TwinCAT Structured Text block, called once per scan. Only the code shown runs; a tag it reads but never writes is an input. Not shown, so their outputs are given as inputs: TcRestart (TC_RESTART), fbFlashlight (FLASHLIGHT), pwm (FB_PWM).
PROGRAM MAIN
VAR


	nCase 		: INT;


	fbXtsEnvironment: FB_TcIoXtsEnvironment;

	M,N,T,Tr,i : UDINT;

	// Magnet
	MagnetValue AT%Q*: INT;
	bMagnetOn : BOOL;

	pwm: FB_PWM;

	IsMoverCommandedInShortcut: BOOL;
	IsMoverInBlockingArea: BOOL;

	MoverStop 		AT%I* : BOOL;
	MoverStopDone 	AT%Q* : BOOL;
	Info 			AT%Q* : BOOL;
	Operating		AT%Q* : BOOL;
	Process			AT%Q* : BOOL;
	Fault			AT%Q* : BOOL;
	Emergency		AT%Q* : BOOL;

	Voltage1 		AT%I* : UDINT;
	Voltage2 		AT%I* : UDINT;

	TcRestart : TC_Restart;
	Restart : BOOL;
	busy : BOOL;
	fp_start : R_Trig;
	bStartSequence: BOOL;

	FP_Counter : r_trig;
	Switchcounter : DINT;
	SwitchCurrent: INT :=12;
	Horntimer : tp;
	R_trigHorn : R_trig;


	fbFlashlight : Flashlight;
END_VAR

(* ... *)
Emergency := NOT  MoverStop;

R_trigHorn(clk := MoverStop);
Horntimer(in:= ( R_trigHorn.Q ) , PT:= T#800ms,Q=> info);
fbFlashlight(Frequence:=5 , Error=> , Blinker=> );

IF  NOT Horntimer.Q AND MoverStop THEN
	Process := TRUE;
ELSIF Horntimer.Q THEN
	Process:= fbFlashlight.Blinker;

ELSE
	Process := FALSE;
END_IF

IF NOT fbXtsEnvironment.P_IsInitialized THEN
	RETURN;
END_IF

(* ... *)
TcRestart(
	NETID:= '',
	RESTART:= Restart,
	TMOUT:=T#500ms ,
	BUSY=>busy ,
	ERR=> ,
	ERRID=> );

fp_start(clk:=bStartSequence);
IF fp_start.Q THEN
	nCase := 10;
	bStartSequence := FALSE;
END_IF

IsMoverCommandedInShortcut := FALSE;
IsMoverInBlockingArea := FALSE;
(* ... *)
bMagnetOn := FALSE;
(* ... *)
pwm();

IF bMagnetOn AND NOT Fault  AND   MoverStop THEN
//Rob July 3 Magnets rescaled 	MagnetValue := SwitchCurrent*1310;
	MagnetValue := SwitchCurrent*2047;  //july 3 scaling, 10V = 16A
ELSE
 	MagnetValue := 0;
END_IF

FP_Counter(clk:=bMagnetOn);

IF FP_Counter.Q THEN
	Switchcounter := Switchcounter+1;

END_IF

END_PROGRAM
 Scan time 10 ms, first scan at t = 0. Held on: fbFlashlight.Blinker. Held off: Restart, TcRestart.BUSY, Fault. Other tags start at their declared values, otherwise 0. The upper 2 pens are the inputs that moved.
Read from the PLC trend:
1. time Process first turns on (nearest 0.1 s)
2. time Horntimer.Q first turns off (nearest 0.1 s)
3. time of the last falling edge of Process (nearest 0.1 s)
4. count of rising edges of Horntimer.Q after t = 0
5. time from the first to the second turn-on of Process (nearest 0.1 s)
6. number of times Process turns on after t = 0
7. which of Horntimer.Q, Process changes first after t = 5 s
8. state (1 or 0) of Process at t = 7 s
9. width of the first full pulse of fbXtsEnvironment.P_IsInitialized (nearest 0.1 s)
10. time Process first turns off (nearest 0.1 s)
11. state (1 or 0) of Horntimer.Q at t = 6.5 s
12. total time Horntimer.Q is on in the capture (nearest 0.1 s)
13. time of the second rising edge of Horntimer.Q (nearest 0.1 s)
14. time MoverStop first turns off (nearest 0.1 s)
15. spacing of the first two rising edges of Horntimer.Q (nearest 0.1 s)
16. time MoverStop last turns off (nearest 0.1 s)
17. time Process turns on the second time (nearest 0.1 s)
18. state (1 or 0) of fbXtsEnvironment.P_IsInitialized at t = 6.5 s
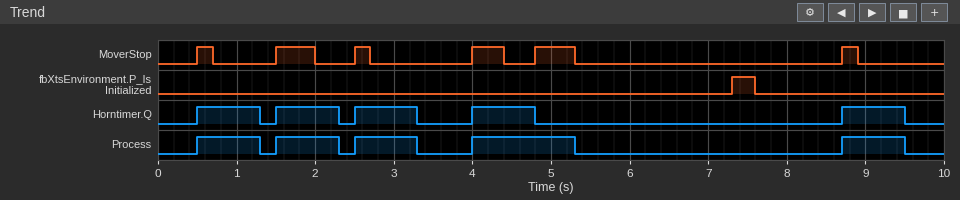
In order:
0.5 s
1.3 s
9.5 s
5
1.0 s
5
Process
0
0.3 s
1.3 s
0
4.0 s
1.5 s
0.7 s
1.0 s
8.9 s
1.5 s
0
